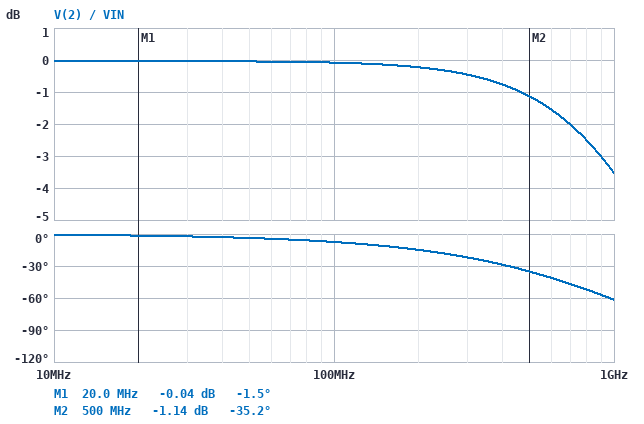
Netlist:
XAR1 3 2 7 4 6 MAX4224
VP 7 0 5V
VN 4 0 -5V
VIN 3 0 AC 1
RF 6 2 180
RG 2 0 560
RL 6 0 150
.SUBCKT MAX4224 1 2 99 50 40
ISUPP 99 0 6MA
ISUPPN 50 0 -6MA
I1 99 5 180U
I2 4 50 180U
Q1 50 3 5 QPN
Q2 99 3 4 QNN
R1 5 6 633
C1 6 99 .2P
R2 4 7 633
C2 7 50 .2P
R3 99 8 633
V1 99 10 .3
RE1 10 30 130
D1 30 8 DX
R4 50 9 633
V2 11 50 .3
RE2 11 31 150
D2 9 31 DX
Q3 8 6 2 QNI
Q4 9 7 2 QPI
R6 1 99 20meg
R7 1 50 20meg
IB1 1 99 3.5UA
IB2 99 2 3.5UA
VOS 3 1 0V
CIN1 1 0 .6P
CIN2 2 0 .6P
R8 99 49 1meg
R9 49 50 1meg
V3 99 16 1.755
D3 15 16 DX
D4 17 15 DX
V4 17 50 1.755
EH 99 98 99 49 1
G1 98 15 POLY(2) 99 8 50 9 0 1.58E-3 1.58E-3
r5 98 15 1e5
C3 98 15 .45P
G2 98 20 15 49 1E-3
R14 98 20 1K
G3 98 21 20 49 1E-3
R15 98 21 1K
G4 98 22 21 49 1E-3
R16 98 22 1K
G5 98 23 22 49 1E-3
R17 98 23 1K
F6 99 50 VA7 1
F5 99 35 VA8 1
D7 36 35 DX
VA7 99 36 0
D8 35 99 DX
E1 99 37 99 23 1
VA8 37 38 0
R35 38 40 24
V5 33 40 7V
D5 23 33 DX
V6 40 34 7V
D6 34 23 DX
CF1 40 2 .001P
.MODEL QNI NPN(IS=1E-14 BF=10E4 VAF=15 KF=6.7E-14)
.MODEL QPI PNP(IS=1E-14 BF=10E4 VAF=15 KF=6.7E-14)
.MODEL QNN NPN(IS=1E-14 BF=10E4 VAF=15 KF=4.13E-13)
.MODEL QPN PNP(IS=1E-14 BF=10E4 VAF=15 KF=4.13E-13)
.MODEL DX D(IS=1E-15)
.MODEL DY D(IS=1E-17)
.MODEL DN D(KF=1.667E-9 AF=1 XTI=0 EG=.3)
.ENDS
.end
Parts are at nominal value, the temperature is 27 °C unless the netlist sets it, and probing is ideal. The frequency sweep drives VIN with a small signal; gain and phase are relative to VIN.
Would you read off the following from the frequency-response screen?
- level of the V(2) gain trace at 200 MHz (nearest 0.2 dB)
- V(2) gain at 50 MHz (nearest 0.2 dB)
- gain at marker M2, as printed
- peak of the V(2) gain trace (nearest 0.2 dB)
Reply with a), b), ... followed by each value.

a) -0.2 dB
b) 0 dB
c) -1.14 dB
d) 0 dB
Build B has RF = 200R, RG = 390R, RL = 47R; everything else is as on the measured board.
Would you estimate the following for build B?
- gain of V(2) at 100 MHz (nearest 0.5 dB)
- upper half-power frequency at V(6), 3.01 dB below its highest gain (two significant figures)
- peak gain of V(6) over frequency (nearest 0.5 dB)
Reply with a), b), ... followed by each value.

a) 0 dB
b) 640 MHz
c) 3.5 dB
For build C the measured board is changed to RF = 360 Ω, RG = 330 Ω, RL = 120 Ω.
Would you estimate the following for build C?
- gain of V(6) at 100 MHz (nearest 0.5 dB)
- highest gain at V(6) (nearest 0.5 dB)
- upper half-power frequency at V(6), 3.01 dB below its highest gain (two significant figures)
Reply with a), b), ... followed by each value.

a) 6.0 dB
b) 6.5 dB
c) 540 MHz
